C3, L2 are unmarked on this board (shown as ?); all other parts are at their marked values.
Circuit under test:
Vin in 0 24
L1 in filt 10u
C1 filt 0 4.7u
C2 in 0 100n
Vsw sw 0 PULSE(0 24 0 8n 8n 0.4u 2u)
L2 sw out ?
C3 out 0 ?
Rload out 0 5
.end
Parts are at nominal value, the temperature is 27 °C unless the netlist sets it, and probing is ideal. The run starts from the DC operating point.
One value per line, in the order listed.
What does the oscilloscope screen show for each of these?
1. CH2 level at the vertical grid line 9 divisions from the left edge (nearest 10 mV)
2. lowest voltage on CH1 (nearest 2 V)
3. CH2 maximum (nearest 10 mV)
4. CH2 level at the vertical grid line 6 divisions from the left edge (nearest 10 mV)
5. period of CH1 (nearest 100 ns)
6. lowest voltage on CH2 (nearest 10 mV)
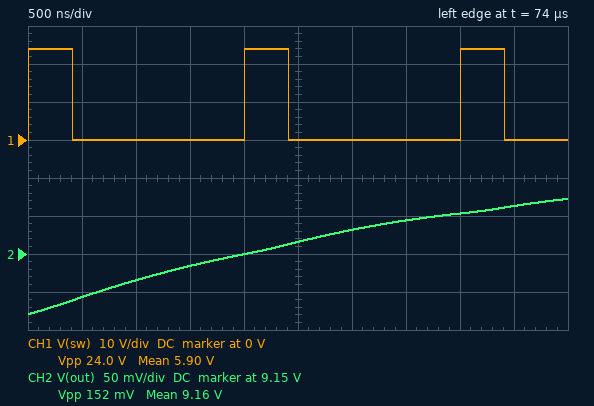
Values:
9.21 V
0 V
9.22 V
9.18 V
2.0 µs
9.07 V
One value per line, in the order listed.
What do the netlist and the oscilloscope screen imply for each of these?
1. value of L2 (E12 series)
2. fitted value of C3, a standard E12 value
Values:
10 µH
68 µF
